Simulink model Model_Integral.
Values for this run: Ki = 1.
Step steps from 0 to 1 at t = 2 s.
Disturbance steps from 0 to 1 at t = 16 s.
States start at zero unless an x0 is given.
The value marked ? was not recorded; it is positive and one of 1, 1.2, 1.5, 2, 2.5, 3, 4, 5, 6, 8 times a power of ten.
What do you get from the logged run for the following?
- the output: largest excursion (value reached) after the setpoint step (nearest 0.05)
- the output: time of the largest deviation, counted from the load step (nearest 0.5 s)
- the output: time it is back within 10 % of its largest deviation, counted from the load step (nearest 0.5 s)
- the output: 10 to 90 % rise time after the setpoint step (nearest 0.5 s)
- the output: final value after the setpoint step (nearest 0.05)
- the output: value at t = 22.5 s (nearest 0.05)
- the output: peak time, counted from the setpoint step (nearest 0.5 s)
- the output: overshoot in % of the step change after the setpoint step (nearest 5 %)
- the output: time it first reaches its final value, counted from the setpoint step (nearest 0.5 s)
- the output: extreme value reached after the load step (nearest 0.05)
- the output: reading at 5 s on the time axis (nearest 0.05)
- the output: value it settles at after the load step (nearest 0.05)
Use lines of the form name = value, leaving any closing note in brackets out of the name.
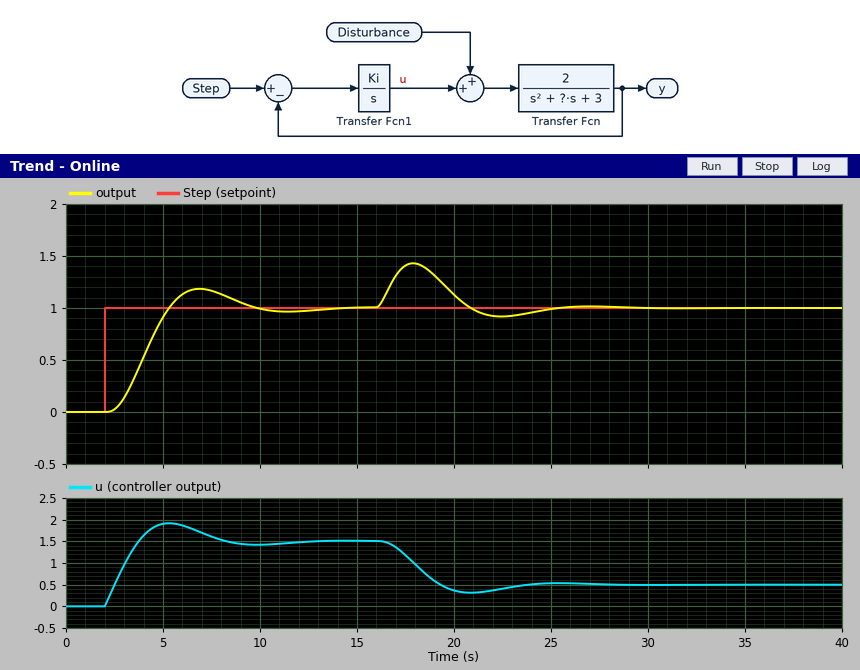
the output: largest excursion (value reached) after the setpoint step = 1.20
the output: time of the largest deviation, counted from the load step = 2.0 s
the output: time it is back within 10 % of its largest deviation, counted from the load step = 8.0 s
the output: 10 to 90 % rise time after the setpoint step = 2.0 s
the output: final value after the setpoint step = 1.00
the output: value at t = 22.5 s = 0.90
the output: peak time, counted from the setpoint step = 5.0 s
the output: overshoot in % of the step change after the setpoint step = 20 %
the output: time it first reaches its final value, counted from the setpoint step = 3.5 s
the output: extreme value reached after the load step = 1.45
the output: reading at 5 s on the time axis = 0.90
the output: value it settles at after the load step = 1.00
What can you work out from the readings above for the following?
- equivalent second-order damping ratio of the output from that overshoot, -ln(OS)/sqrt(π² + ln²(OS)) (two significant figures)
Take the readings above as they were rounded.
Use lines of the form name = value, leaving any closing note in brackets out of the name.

equivalent second-order damping ratio of the output from that overshoot, -ln(OS)/sqrt(π² + ln²(OS)) = 0.46
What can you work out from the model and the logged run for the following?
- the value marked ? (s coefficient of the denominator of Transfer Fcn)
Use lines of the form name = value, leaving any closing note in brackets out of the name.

the value marked ? = 4
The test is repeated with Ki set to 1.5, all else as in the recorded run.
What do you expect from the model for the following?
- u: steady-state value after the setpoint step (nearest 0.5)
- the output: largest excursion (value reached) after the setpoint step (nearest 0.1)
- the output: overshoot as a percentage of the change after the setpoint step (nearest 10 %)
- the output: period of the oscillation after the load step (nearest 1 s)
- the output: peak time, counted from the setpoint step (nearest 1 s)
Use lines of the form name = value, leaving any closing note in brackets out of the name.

u: steady-state value after the setpoint step = 1.5
the output: largest excursion (value reached) after the setpoint step = 1.3
the output: overshoot as a percentage of the change after the setpoint step = 30 %
the output: period of the oscillation after the load step = 7 s
the output: peak time, counted from the setpoint step = 4 s
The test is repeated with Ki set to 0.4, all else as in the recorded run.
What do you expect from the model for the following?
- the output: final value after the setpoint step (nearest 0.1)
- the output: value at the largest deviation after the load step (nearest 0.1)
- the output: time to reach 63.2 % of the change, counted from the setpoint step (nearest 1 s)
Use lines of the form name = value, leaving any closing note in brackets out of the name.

the output: final value after the setpoint step = 1.0
the output: value at the largest deviation after the load step = 1.5
the output: time to reach 63.2 % of the change, counted from the setpoint step = 4 s
